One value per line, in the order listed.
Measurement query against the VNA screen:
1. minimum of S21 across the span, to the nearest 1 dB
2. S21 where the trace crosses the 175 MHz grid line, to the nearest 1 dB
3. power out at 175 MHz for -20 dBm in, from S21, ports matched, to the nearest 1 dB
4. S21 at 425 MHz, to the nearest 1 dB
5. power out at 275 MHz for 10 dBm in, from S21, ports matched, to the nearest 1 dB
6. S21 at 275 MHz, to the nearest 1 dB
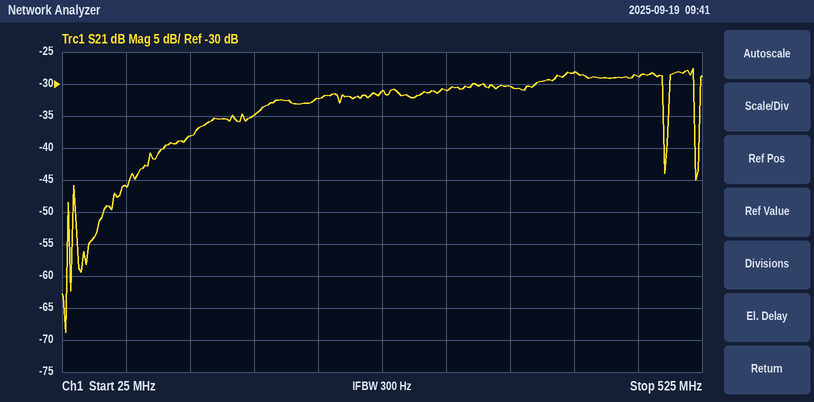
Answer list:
-69 dB
-35 dB
-55 dBm
-28 dB
-21 dBm
-31 dB
